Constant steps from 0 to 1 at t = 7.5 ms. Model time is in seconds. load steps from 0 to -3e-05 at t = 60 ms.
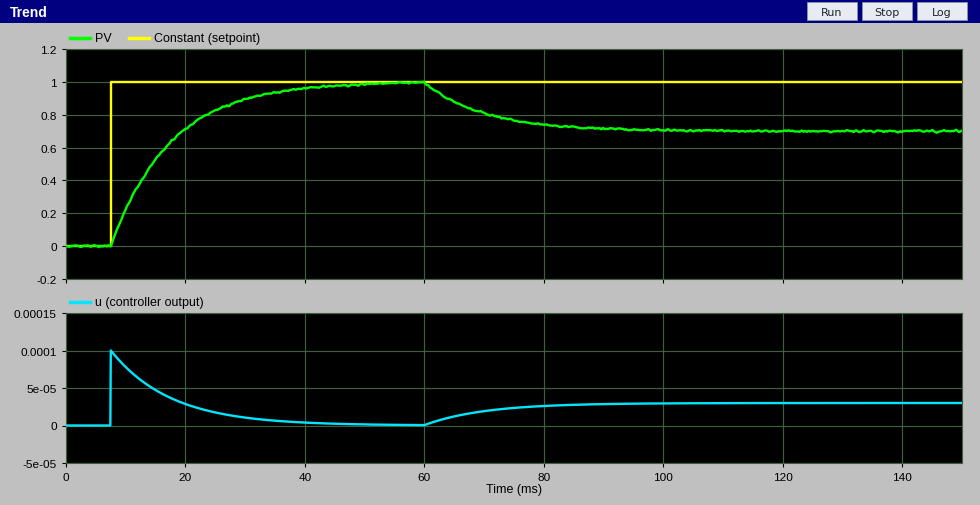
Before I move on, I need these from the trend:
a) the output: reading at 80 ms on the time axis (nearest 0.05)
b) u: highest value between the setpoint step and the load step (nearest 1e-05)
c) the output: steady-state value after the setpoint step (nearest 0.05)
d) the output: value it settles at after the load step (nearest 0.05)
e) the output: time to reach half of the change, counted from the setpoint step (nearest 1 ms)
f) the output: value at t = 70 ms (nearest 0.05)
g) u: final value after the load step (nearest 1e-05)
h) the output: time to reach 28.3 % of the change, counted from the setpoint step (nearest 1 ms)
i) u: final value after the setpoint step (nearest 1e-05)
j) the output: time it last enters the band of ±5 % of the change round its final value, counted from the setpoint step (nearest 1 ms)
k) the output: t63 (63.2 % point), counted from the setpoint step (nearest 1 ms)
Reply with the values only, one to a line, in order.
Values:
0.75
0.00010
1.00
0.70
7 ms
0.80
0.00003
3 ms
0.00000
30 ms
10 ms
